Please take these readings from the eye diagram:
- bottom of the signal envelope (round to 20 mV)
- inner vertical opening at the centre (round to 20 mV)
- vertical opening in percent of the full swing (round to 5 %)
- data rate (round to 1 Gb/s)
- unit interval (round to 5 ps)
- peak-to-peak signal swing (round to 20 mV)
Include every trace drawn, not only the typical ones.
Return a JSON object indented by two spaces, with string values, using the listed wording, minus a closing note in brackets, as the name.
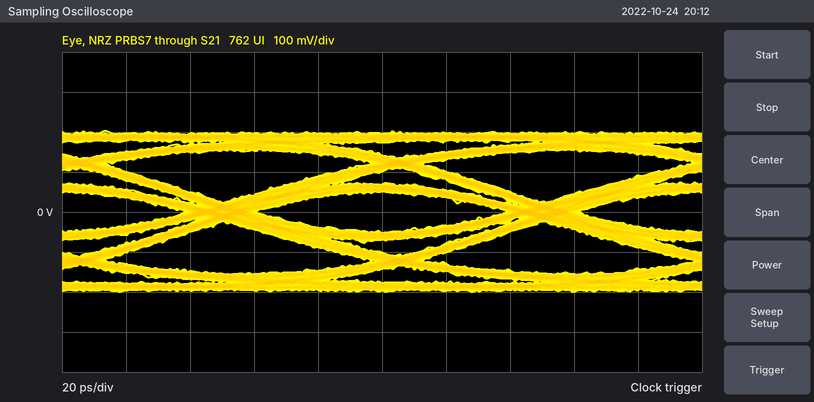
{
  "bottom of the signal envelope": "-200 mV",
  "inner vertical opening at the centre": "100 mV",
  "vertical opening in percent of the full swing": "25 %",
  "data rate": "10 Gb/s",
  "unit interval": "100 ps",
  "peak-to-peak signal swing": "400 mV"
}
